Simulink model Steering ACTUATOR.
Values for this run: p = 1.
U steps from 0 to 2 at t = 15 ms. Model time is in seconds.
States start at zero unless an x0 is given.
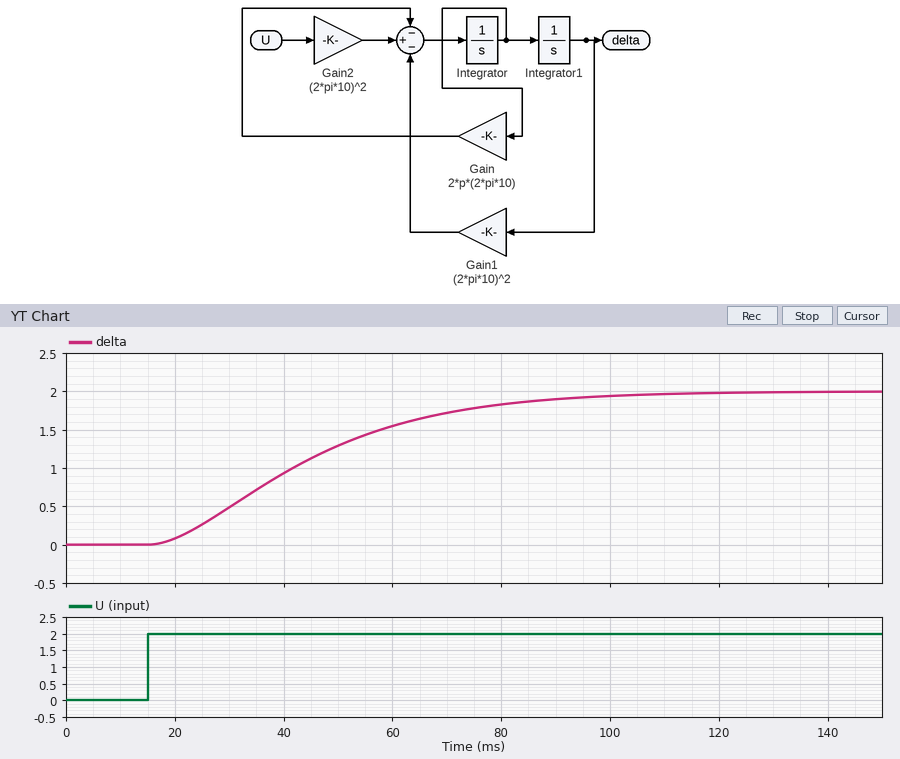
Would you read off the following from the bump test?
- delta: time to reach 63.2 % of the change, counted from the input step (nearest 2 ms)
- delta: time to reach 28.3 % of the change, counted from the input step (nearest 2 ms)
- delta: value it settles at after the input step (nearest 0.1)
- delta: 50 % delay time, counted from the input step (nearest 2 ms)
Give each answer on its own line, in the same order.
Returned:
34 ms
16 ms
2.0
26 ms
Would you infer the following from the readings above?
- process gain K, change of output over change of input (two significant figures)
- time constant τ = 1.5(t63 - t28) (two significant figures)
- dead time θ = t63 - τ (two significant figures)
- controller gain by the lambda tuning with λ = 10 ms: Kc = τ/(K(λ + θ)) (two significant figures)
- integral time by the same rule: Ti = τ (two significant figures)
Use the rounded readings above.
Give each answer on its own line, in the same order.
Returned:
1.0
27 ms
7.0 ms
1.6
27 ms
